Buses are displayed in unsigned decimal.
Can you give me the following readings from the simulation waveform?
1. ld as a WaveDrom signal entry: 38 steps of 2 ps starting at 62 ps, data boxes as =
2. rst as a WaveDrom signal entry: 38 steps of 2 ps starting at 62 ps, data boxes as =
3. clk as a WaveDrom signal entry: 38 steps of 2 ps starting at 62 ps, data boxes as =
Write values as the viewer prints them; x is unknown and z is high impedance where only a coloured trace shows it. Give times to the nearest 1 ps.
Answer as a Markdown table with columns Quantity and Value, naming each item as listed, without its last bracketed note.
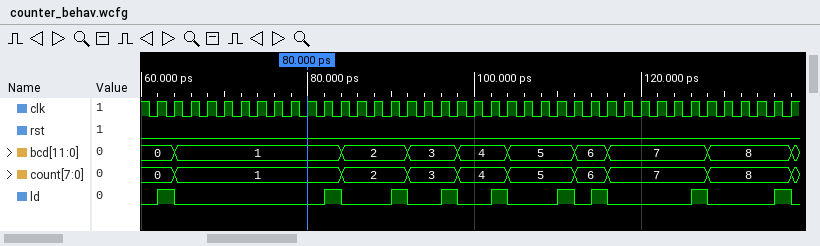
| Quantity | Value |
|---|---|
| ld as a WaveDrom signal entry: 38 steps of 2 ps starting at 62 ps, data boxes as = | {name: 'ld', wave: '10........10..10.10.10..1010....10...1'} |
| rst as a WaveDrom signal entry: 38 steps of 2 ps starting at 62 ps, data boxes as = | {name: 'rst', wave: '0.....................................'} |
| clk as a WaveDrom signal entry: 38 steps of 2 ps starting at 62 ps, data boxes as = | {name: 'clk', wave: 'p.....................................'} |
